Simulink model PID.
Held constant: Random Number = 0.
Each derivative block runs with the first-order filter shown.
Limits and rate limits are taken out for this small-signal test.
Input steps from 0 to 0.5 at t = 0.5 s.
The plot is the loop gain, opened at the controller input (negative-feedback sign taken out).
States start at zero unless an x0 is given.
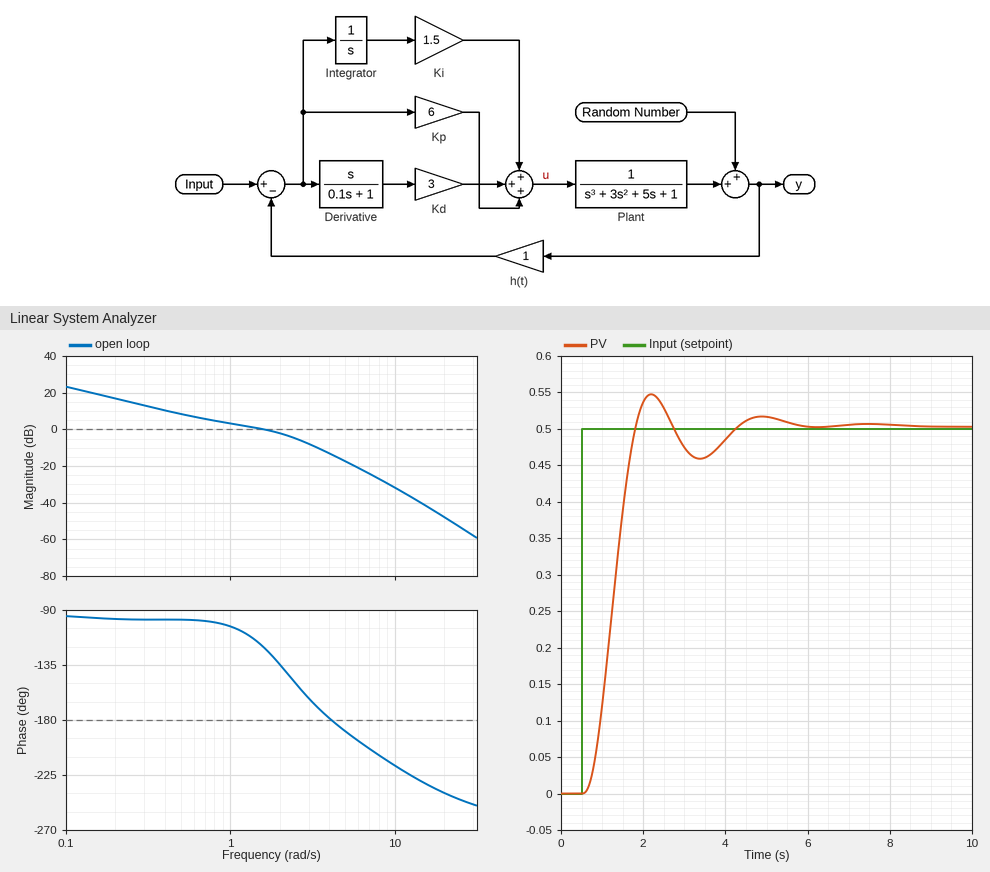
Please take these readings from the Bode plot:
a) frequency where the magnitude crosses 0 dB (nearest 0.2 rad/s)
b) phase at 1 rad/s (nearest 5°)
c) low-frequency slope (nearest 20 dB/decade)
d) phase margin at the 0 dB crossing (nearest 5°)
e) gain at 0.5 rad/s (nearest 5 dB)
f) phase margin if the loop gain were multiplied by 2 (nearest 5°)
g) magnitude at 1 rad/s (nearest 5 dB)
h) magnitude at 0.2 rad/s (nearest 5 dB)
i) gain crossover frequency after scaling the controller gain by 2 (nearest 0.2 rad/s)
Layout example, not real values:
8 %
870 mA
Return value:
1.6 rad/s
-105°
-20 dB/decade
60°
10 dB
25°
5 dB
15 dB
2.6 rad/s
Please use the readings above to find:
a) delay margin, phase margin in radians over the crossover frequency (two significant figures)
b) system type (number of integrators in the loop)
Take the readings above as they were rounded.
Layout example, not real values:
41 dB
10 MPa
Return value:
0.65 s
1
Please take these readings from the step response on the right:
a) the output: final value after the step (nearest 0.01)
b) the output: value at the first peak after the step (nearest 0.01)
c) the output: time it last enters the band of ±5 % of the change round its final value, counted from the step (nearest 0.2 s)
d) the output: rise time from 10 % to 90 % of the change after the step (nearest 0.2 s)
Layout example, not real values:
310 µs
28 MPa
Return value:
0.50
0.55
3.4 s
0.8 s
